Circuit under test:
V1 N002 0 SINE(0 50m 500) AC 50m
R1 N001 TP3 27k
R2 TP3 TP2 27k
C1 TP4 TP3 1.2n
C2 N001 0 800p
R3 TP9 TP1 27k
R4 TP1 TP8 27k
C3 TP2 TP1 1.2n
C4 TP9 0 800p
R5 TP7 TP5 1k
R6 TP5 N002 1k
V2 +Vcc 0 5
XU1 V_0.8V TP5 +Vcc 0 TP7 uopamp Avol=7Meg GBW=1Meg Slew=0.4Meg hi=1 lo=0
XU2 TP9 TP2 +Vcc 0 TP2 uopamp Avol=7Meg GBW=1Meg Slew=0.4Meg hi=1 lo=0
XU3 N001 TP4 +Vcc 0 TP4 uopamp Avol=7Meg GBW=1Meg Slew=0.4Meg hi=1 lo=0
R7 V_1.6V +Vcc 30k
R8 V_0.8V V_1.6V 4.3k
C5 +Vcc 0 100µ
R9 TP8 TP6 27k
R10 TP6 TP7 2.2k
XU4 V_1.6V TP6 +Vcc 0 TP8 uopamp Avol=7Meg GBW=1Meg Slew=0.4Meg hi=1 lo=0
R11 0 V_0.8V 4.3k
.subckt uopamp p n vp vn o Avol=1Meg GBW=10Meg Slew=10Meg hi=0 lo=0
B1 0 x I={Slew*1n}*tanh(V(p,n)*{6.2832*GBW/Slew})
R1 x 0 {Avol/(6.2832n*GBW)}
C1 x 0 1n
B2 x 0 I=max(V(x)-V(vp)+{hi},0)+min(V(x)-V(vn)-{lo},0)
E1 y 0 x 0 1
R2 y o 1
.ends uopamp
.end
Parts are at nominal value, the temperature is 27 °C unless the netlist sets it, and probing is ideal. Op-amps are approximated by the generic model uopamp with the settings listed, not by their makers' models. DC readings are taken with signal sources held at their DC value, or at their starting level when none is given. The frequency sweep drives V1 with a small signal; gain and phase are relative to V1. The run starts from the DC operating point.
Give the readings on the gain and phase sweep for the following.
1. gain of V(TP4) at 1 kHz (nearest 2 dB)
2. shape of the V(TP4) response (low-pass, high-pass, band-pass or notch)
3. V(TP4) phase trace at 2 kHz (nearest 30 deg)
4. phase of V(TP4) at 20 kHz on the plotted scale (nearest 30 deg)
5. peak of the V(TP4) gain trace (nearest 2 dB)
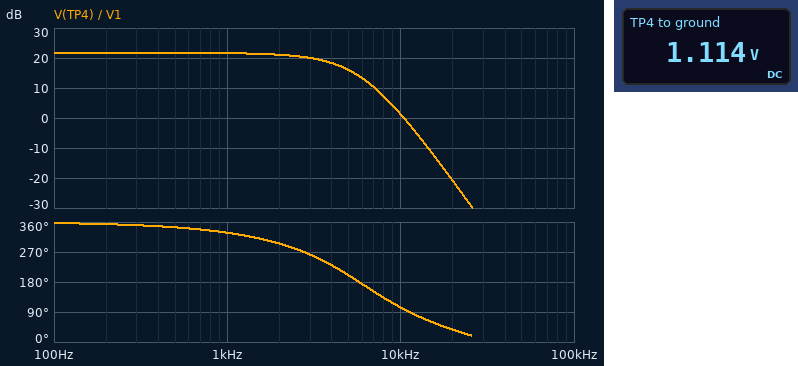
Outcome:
22 dB
low-pass
300 deg
30 deg
22 dB
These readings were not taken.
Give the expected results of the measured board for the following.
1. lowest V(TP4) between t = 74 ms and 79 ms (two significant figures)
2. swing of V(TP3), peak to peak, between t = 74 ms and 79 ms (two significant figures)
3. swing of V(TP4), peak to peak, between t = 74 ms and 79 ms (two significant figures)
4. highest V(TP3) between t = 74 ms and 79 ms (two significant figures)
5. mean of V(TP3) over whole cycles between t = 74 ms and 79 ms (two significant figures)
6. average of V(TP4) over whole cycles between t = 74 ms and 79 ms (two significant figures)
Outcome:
500 mV
1.2 V
1.2 V
1.7 V
1.1 V
1.1 V
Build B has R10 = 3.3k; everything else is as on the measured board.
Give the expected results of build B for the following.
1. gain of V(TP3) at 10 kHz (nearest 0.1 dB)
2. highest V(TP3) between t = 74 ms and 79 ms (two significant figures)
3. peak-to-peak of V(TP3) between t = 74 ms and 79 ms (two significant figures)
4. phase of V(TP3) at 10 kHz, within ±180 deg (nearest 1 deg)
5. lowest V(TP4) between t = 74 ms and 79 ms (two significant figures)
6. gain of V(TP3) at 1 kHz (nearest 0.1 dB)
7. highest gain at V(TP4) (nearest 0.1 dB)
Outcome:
2.3 dB
1.5 V
820 mV
160 deg
710 mV
18.2 dB
18.3 dB
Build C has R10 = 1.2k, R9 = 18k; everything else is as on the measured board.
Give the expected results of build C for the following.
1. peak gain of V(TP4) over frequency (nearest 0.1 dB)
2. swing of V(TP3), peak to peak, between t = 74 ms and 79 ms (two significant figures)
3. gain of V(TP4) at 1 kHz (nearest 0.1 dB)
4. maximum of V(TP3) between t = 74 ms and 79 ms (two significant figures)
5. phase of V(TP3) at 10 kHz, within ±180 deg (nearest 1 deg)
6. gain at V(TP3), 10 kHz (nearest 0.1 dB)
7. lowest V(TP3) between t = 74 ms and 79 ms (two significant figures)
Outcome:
23.5 dB
1.5 V
23.4 dB
1.9 V
156 deg
7.5 dB
370 mV
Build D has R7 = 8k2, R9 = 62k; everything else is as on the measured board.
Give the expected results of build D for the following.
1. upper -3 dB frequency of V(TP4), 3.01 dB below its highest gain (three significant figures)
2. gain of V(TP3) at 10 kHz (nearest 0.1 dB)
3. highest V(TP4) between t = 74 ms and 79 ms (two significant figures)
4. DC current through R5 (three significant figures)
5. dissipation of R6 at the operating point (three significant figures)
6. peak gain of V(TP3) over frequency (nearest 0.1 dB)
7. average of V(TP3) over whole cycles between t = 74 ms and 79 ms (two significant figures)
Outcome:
3.75 kHz
12.7 dB
4.0 V
1.28 mA
1.64 mW
29.0 dB
2.6 V
